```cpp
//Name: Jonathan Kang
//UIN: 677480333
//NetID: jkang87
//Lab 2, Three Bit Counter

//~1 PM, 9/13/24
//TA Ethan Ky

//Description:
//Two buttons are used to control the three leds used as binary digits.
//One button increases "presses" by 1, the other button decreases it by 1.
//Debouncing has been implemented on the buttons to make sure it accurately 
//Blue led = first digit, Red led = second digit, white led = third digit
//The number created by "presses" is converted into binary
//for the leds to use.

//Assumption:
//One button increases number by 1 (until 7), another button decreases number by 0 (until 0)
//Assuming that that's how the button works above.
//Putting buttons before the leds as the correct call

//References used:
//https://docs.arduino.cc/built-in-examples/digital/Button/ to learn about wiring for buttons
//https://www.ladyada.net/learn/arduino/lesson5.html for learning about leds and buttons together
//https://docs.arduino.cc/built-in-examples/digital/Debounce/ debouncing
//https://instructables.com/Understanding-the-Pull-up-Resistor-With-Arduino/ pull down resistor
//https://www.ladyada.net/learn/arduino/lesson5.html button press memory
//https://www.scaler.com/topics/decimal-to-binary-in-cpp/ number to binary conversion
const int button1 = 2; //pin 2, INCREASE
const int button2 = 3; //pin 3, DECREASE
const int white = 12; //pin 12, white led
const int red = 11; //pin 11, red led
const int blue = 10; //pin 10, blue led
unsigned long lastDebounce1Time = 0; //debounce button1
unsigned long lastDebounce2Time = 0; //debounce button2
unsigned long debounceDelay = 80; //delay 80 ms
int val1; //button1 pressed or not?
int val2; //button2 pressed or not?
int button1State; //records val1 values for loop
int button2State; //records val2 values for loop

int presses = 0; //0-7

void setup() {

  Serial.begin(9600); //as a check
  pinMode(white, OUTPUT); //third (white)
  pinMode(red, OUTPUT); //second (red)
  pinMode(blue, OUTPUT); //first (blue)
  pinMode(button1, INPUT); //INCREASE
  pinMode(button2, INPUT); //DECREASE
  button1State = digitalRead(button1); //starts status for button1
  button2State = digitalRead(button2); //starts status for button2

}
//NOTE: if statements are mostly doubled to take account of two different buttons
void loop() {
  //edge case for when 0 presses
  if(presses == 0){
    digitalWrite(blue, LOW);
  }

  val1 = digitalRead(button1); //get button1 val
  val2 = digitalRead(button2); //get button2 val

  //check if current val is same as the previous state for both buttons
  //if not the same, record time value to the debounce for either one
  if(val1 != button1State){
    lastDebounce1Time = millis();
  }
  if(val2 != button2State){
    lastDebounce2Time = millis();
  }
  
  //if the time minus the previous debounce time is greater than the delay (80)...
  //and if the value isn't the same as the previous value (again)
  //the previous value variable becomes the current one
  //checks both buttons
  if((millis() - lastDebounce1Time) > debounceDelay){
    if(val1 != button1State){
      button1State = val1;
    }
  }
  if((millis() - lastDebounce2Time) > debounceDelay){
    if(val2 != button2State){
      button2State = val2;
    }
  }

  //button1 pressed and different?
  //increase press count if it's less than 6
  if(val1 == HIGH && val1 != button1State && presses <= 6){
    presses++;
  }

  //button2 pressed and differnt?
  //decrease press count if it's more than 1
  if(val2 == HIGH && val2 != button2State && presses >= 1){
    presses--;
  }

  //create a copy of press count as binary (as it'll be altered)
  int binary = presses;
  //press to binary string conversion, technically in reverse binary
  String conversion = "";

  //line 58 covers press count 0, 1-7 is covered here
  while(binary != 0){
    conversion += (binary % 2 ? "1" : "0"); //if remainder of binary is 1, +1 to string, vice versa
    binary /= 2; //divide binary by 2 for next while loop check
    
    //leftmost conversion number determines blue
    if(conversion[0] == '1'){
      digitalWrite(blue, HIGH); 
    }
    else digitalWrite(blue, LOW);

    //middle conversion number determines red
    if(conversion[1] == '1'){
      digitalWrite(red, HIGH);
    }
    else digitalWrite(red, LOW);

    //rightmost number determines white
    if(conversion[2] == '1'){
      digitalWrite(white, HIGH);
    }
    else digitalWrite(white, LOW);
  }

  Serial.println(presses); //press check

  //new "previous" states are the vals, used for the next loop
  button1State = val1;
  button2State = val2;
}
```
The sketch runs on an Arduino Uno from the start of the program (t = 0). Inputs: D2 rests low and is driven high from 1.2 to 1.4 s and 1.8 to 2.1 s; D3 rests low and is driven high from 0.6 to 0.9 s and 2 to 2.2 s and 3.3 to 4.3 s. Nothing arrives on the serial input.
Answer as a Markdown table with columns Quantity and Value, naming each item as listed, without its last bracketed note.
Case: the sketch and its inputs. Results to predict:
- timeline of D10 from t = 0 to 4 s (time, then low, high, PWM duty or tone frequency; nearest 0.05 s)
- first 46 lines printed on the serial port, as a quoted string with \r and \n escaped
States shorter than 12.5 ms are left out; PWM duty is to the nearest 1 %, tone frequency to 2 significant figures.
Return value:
| Quantity | Value |
|---|---|
| timeline of D10 from t = 0 to 4 s | 0 s low; 1.2 s high; 1.8 s low; 2 s high; 3.3 s low |
| first 46 lines printed on the serial port, as a quoted string with \r and \n escaped | "0\r\n0\r\n0\r\n0\r\n0\r\n0\r\n0\r\n0\r\n0\r\n0\r\n0\r\n0\r\n0\r\n0\r\n0\r\n0\r\n0\r\n0\r\n0\r\n0\r\n0\r\n0\r\n0\r\n0\r\n0\r\n0\r\n0\r\n0\r\n0\r\n0\r\n0\r\n0\r\n0\r\n0\r\n0\r\n0\r\n0\r\n0\r\n0\r\n0\r\n0\r\n0\r\n0\r\n0\r\n0\r\n0\r\n" |
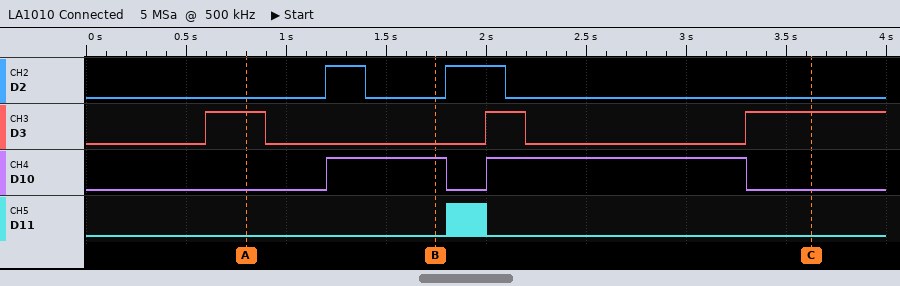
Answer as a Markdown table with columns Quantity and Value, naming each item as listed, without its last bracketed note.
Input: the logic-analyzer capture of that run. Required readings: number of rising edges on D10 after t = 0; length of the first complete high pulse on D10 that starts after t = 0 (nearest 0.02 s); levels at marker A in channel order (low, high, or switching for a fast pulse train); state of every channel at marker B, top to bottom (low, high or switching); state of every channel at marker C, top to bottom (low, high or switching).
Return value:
| Quantity | Value |
|---|---|
| number of rising edges on D10 after t = 0 | 2 |
| length of the first complete high pulse on D10 that starts after t = 0 | 0.60 s |
| levels at marker A in channel order | D2 low, D3 high, D10 low, D11 low |
| state of every channel at marker B, top to bottom | D2 low, D3 low, D10 high, D11 low |
| state of every channel at marker C, top to bottom | D2 low, D3 high, D10 low, D11 low |
